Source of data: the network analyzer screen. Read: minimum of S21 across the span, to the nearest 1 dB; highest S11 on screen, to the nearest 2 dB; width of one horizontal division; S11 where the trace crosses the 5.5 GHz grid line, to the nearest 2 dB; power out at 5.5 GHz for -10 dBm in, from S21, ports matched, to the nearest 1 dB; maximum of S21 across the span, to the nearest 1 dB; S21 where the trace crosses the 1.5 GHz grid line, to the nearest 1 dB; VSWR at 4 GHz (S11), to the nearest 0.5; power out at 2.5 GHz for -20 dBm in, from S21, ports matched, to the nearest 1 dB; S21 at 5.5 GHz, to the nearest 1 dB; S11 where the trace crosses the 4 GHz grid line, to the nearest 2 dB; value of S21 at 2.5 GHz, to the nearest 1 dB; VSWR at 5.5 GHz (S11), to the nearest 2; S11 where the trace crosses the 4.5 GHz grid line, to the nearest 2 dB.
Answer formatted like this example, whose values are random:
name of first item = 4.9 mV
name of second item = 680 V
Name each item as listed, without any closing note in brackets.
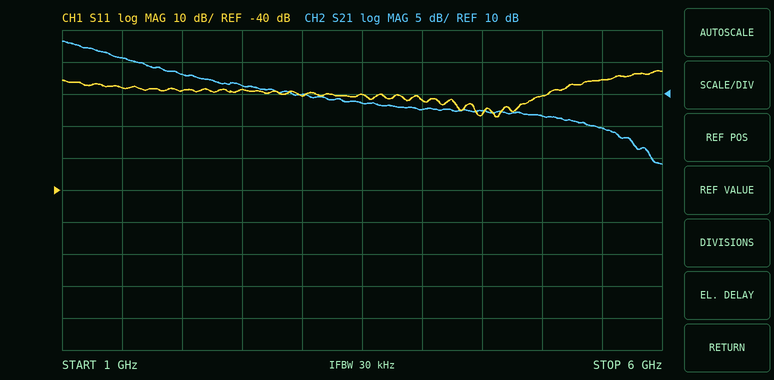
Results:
minimum of S21 across the span, to the nearest 1 dB = -1 dB
highest S11 on screen, to the nearest 2 dB = -2 dB
width of one horizontal division = 500 MHz
S11 where the trace crosses the 5.5 GHz grid line, to the nearest 2 dB = -6 dB
power out at 5.5 GHz for -10 dBm in, from S21, ports matched, to the nearest 1 dB = -5 dBm
maximum of S21 across the span, to the nearest 1 dB = 18 dB
S21 where the trace crosses the 1.5 GHz grid line, to the nearest 1 dB = 16 dB
VSWR at 4 GHz (S11), to the nearest 0.5 = 1.5
power out at 2.5 GHz for -20 dBm in, from S21, ports matched, to the nearest 1 dB = -9 dBm
S21 at 5.5 GHz, to the nearest 1 dB = 5 dB
S11 where the trace crosses the 4 GHz grid line, to the nearest 2 dB = -12 dB
value of S21 at 2.5 GHz, to the nearest 1 dB = 11 dB
VSWR at 5.5 GHz (S11), to the nearest 2 = 4
S11 where the trace crosses the 4.5 GHz grid line, to the nearest 2 dB = -16 dB
